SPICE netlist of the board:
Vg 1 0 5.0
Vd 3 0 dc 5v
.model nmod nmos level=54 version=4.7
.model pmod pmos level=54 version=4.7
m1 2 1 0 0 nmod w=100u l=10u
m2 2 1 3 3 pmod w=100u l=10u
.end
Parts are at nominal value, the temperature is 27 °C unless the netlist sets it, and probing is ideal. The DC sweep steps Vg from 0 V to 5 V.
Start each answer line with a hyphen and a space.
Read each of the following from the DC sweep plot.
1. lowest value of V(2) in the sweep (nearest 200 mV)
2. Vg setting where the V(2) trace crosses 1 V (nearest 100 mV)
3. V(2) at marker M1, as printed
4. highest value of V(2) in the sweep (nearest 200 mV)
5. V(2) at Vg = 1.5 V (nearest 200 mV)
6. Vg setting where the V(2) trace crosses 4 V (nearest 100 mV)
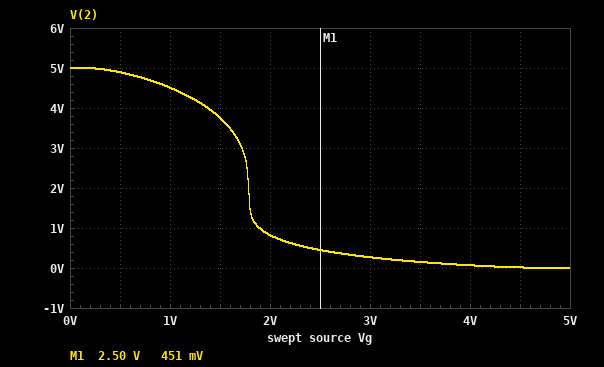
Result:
- 0 V
- 1.9 V
- 451 mV
- 5.0 V
- 3.8 V
- 1.4 V
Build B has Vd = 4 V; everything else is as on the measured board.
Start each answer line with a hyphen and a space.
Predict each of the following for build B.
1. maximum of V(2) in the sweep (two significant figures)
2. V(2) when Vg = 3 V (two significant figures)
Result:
- 4.0 V
- 71 mV
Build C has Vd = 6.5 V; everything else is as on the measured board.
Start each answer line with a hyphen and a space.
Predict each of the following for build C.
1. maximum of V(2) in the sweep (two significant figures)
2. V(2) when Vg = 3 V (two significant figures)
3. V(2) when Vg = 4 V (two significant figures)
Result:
- 6.5 V
- 720 mV
- 370 mV
